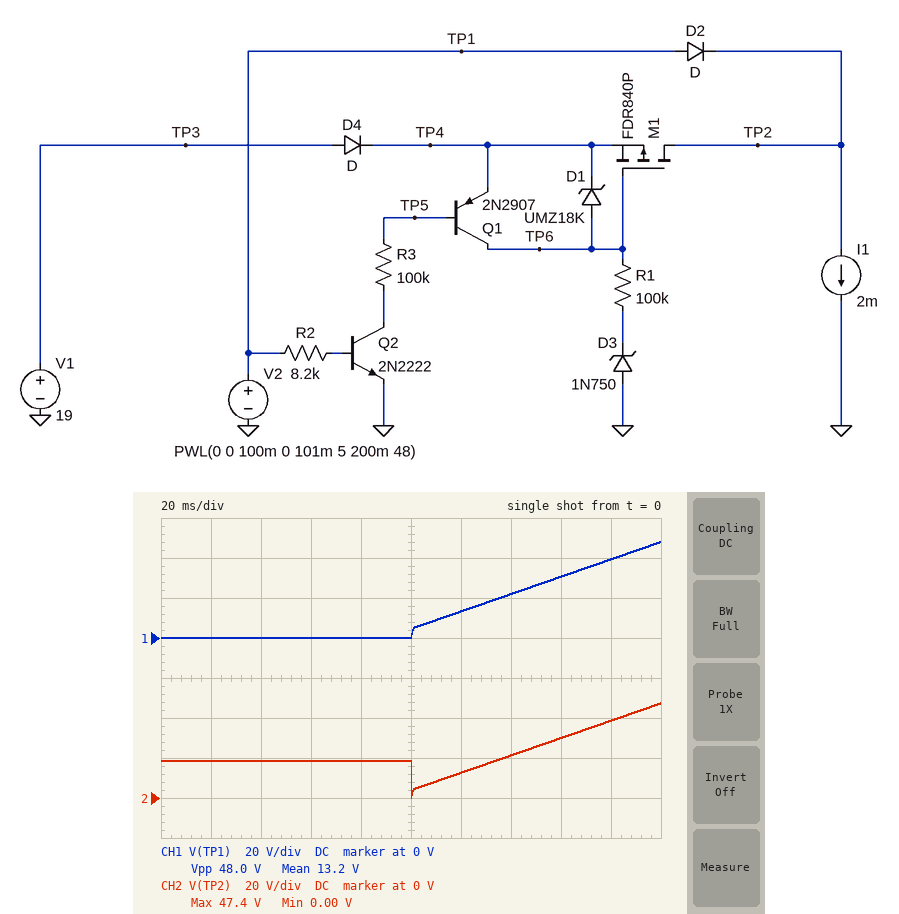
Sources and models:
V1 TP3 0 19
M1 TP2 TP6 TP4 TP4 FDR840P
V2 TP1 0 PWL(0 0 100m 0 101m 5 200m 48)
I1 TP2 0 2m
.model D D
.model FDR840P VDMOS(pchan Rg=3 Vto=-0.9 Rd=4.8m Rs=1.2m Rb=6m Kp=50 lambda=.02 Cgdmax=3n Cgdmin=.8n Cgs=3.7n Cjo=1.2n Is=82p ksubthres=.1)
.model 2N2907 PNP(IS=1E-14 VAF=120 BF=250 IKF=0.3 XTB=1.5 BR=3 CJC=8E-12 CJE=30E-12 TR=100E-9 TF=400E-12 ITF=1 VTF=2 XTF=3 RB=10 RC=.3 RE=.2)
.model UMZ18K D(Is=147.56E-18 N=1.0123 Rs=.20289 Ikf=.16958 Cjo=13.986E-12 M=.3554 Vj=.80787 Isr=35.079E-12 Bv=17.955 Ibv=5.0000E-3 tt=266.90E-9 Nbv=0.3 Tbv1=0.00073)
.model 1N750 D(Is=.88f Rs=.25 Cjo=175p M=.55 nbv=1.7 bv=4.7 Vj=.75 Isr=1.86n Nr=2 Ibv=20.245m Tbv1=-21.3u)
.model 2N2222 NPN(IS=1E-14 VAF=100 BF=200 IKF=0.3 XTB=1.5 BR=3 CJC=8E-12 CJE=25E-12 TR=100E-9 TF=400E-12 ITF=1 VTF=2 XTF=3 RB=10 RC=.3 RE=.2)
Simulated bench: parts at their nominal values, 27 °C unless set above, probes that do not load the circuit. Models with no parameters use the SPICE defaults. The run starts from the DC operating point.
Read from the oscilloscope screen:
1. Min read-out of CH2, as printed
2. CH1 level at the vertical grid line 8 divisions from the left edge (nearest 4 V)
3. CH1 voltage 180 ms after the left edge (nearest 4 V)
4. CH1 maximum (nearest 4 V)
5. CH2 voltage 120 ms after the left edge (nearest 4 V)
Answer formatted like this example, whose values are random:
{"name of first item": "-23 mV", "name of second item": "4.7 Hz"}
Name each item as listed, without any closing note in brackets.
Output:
{"Min read-out of CH2, as printed": "0.00 V", "CH1 level at the vertical grid line 8 divisions from the left edge": "32 V", "CH1 voltage 180 ms after the left edge": "40 V", "CH1 maximum": "48 V", "CH2 voltage 120 ms after the left edge": "12 V"}
